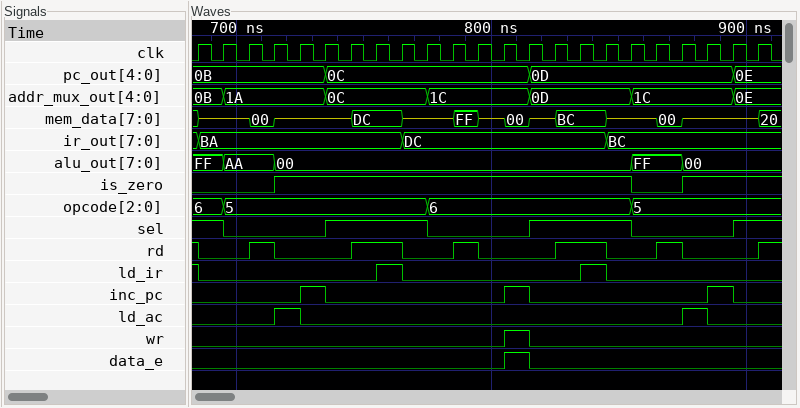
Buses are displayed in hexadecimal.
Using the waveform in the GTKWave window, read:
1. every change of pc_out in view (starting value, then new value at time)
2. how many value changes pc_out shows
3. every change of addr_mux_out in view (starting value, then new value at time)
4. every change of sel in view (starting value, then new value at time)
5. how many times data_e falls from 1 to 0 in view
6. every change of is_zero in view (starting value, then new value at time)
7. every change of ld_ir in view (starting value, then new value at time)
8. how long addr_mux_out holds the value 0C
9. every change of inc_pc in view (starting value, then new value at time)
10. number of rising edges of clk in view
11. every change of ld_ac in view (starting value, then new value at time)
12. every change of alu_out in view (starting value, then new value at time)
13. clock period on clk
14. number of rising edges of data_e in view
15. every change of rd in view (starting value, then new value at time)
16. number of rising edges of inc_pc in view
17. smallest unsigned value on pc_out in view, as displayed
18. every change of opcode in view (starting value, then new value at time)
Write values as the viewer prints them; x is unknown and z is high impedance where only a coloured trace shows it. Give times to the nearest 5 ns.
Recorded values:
0B, 0C at 735 ns, 0D at 815 ns, 0E at 895 ns
3
0B, 1A at 695 ns, 0C at 735 ns, 1C at 775 ns, 0D at 815 ns, 1C at 855 ns, 0E at 895 ns
1, 0 at 695 ns, 1 at 735 ns, 0 at 775 ns, 1 at 815 ns, 0 at 855 ns, 1 at 895 ns
1
0, 1 at 715 ns, 0 at 855 ns, 1 at 875 ns
1, 0 at 685 ns, 1 at 755 ns, 0 at 765 ns, 1 at 835 ns, 0 at 845 ns
40 ns
0, 1 at 725 ns, 0 at 735 ns, 1 at 805 ns, 0 at 815 ns, 1 at 885 ns, 0 at 895 ns
23
0, 1 at 715 ns, 0 at 725 ns, 1 at 875 ns, 0 at 885 ns
FF, AA at 695 ns, 00 at 715 ns, FF at 855 ns, 00 at 875 ns
10 ns
1
1, 0 at 685 ns, 1 at 705 ns, 0 at 715 ns, 1 at 745 ns, 0 at 765 ns, 1 at 785 ns, 0 at 795 ns, 1 at 825 ns, 0 at 845 ns, 1 at 865 ns, 0 at 875 ns, 1 at 905 ns
3
0B
6, 5 at 695 ns, 6 at 775 ns, 5 at 855 ns
